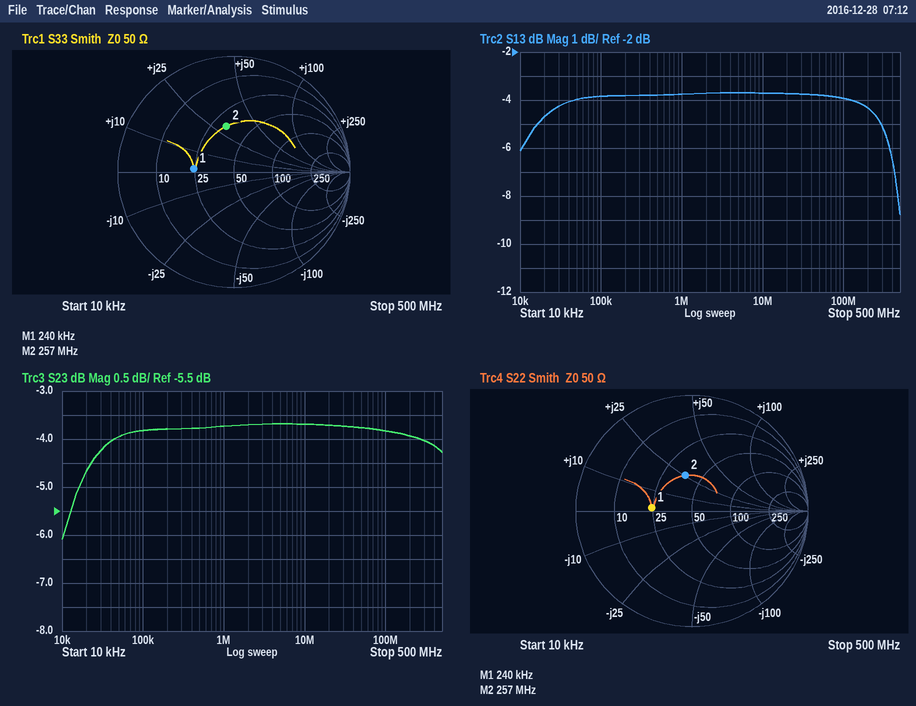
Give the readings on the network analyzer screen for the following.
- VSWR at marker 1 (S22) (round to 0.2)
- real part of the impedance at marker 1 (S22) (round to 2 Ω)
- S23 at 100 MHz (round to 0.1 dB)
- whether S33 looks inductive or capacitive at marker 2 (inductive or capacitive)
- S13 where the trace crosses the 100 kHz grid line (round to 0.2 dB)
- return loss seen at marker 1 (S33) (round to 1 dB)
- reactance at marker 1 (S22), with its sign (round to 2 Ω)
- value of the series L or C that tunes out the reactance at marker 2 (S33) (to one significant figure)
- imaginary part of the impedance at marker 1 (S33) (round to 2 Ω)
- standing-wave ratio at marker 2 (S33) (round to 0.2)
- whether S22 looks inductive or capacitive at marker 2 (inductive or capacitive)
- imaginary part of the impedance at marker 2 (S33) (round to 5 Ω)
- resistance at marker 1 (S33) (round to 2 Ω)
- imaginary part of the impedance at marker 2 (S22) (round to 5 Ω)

2.0
24 Ω
-3.8 dB
inductive
-3.8 dB
9 dB
+2 Ω
20 pF
+2 Ω
2.4
inductive
+30 Ω
24 Ω
+25 Ω
